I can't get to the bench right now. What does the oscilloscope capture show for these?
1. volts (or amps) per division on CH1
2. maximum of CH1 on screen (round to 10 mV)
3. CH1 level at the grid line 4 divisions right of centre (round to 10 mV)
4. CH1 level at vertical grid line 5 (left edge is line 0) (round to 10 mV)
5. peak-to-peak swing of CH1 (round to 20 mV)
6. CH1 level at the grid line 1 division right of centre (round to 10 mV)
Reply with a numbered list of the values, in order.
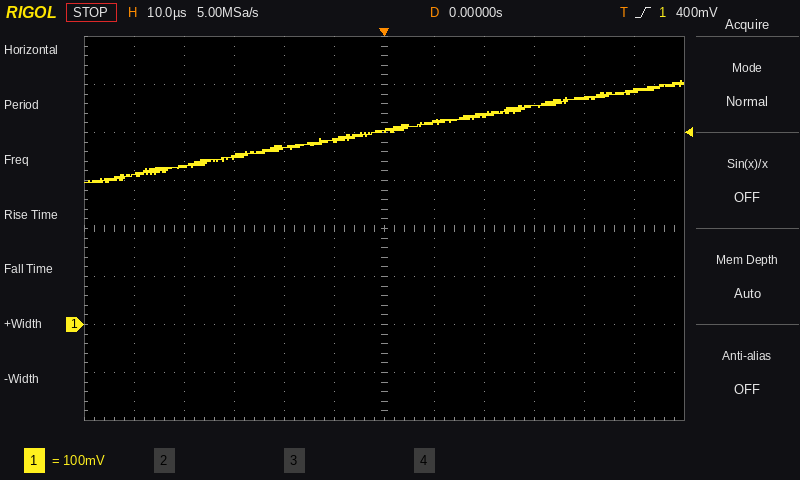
1. 100 mV
2. 510 mV
3. 470 mV
4. 380 mV
5. 220 mV
6. 420 mV
